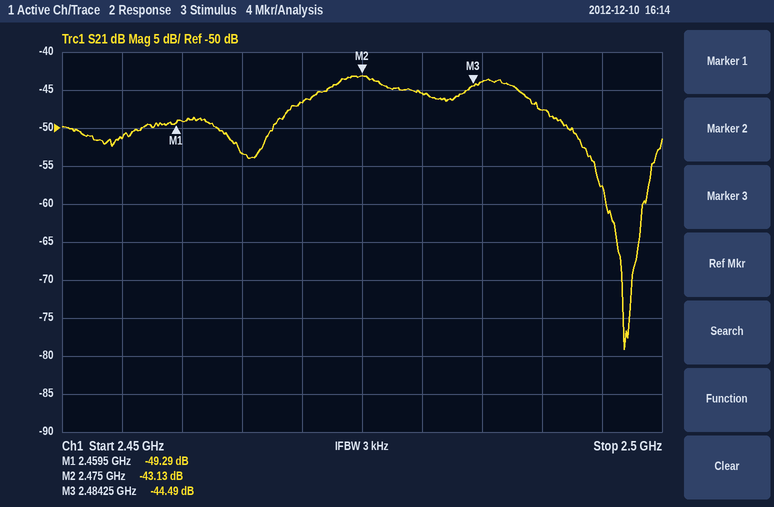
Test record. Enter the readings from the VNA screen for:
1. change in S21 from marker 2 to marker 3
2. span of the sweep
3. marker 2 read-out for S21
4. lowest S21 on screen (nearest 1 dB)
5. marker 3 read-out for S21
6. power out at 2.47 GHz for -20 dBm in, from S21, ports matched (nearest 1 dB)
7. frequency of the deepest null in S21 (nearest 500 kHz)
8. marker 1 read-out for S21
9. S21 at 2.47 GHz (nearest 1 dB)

-1.36 dB
50 MHz
-43.13 dB
-79 dB
-44.49 dB
-67 dBm
2.4970 GHz
-49.29 dB
-47 dB
